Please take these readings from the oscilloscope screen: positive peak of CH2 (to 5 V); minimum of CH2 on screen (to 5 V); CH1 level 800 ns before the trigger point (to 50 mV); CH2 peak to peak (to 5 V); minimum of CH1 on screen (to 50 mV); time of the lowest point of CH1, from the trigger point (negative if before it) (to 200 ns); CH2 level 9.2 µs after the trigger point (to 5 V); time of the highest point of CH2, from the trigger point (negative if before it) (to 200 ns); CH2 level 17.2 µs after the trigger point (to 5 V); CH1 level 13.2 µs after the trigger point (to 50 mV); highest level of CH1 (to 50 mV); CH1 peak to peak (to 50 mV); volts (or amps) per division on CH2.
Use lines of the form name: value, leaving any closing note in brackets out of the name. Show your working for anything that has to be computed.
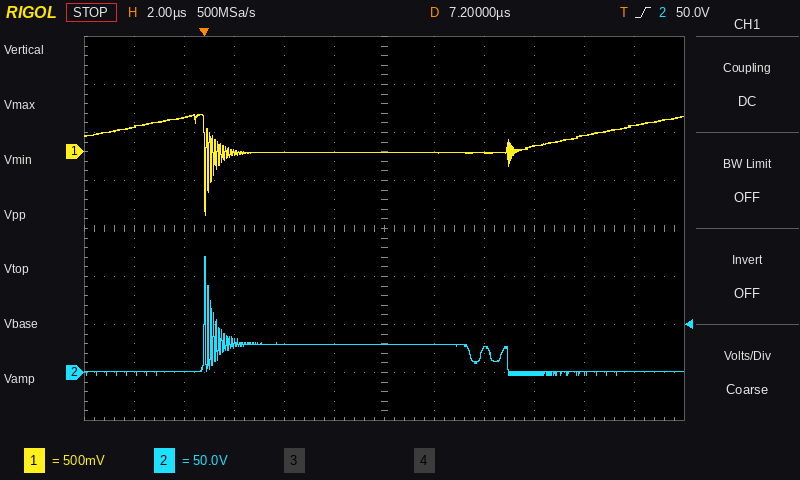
positive peak of CH2: 120 V
minimum of CH2 on screen: -5 V
CH1 level 800 ns before the trigger point: 350 mV
CH2 peak to peak: 120 V − (-5 V) = 125 V
minimum of CH1 on screen: -650 mV
time of the lowest point of CH1, from the trigger point (negative if before it): 0.0 µs
CH2 level 9.2 µs after the trigger point: 30 V
time of the highest point of CH2, from the trigger point (negative if before it): 0.0 µs
CH2 level 17.2 µs after the trigger point: 0 V
CH1 level 13.2 µs after the trigger point: 50 mV
highest level of CH1: 400 mV
CH1 peak to peak: 400 mV − (-650 mV) = 1.05 V
volts (or amps) per division on CH2: 50 V
